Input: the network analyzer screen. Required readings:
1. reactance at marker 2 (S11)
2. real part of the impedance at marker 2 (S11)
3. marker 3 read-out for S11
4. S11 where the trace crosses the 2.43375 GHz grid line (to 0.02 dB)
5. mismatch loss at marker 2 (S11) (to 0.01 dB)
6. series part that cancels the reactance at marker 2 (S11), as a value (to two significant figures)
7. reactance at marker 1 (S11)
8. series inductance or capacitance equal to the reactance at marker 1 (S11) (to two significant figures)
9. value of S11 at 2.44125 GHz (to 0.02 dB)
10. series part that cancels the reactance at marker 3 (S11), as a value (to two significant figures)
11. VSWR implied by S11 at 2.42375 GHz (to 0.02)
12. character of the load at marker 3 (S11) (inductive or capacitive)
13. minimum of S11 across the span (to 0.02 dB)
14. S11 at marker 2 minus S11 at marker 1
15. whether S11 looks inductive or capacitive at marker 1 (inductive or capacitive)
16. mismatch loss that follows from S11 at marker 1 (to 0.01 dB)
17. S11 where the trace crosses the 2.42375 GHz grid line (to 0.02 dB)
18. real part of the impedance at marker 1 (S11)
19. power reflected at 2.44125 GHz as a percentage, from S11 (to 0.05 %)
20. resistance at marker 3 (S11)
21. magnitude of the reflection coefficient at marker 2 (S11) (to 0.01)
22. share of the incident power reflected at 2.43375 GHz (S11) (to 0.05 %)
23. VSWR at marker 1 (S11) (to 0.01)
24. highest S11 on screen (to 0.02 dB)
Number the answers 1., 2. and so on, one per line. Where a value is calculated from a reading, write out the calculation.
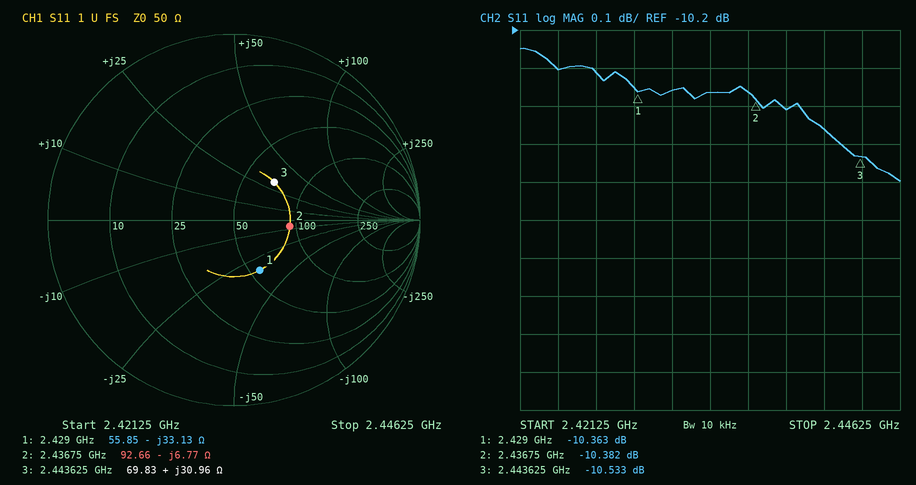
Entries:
1. -6.77 Ω
2. 92.66 Ω
3. -10.533 dB
4. -10.36 dB
5. −10 log10(1 − 10^(-10.382/10)) ≈ 0.42 dB
6. L = 6.77 Ω/(2π × 2.43675 GHz) ≈ 442 pH, so 440 pH to two significant figures
7. -33.13 Ω
8. C = 1/(2π × 2.429 GHz × 33.13 Ω) ≈ 2.0 pF
9. -10.46 dB
10. C = 1/(2π × 2.443625 GHz × 30.96 Ω) ≈ 2.1 pF
11. |Γ| = 10^(-10.3/20) = 0.3055; VSWR = (1 + 0.3055)/(1 − 0.3055) ≈ 1.88
12. inductive
13. -10.60 dB
14. -10.382 − (-10.363) = -0.019 dB
15. capacitive
16. −10 log10(1 − 10^(-10.363/10)) ≈ 0.42 dB
17. -10.30 dB
18. 55.85 Ω
19. 10^(-10.46/10) ≈ 8.99 %, so 9.00 % to the nearest 0.05 %
20. 69.83 Ω
21. 0.30
22. 10^(-10.36/10) ≈ 9.20 %
23. 1.87
24. -10.24 dB
